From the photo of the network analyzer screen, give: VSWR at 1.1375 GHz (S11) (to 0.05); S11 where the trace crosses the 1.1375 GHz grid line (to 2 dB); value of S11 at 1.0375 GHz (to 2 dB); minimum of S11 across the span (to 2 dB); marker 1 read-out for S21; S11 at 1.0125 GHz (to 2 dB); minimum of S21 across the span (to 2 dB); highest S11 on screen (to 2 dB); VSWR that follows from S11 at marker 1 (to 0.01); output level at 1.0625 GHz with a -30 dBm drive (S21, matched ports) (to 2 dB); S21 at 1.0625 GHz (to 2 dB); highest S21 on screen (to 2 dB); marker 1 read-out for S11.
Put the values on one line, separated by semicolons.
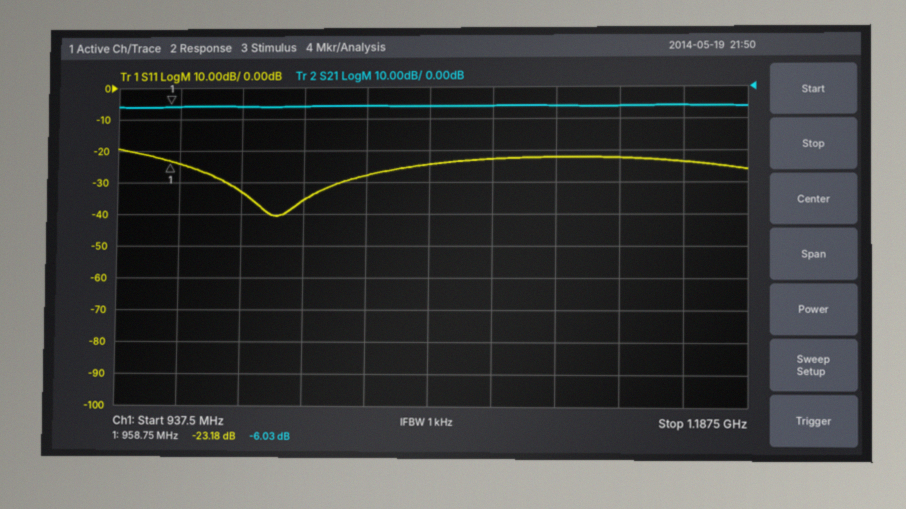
1.15; -22 dB; -28 dB; -40 dB; -6.03 dB; -36 dB; -6 dB; -20 dB; 1.15; -36 dBm; -6 dB; -6 dB; -23.18 dB
